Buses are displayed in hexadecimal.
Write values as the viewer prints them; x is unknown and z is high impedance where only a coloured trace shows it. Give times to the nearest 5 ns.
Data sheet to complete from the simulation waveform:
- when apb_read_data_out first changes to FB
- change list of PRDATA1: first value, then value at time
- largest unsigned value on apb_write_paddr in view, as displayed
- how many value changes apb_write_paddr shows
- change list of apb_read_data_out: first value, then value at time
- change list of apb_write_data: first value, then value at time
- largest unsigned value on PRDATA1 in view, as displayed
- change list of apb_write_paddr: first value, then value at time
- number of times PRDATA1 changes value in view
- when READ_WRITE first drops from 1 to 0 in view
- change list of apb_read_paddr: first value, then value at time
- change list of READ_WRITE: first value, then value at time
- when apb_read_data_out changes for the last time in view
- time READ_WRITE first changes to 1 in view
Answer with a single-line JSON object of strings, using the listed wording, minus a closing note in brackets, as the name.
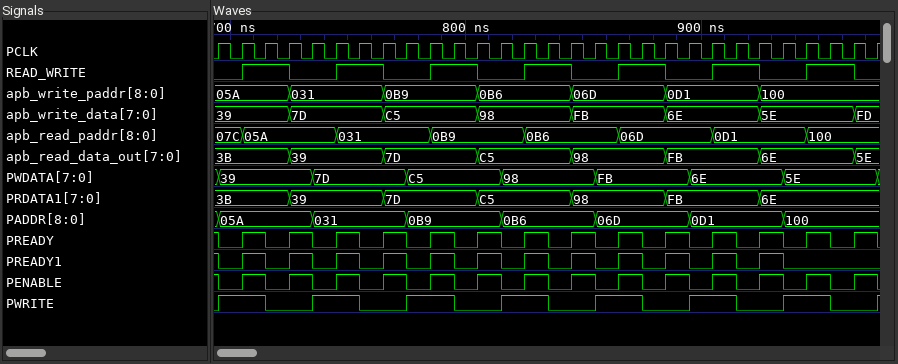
{"when apb_read_data_out first changes to FB": "885 ns", "change list of PRDATA1: first value, then value at time": "3B, 39 at 725 ns, 7D at 765 ns, C5 at 805 ns, 98 at 845 ns, FB at 885 ns, 6E at 925 ns", "largest unsigned value on apb_write_paddr in view, as displayed": "100", "how many value changes apb_write_paddr shows": "6", "change list of apb_read_data_out: first value, then value at time": "3B, 39 at 725 ns, 7D at 765 ns, C5 at 805 ns, 98 at 845 ns, FB at 885 ns, 6E at 925 ns, 5E at 965 ns", "change list of apb_write_data: first value, then value at time": "39, 7D at 725 ns, C5 at 765 ns, 98 at 805 ns, FB at 845 ns, 6E at 885 ns, 5E at 925 ns, FD at 965 ns", "largest unsigned value on PRDATA1 in view, as displayed": "FB", "change list of apb_write_paddr: first value, then value at time": "05A, 031 at 725 ns, 0B9 at 765 ns, 0B6 at 805 ns, 06D at 845 ns, 0D1 at 885 ns, 100 at 925 ns", "number of times PRDATA1 changes value in view": "6", "when READ_WRITE first drops from 1 to 0 in view": "725 ns", "change list of apb_read_paddr: first value, then value at time": "07C, 05A at 705 ns, 031 at 745 ns, 0B9 at 785 ns, 0B6 at 825 ns, 06D at 865 ns, 0D1 at 905 ns, 100 at 945 ns", "change list of READ_WRITE: first value, then value at time": "0, 1 at 705 ns, 0 at 725 ns, 1 at 745 ns, 0 at 765 ns, 1 at 785 ns, 0 at 805 ns, 1 at 825 ns, 0 at 845 ns, 1 at 865 ns, 0 at 885 ns, 1 at 905 ns, 0 at 925 ns, 1 at 945 ns, 0 at 965 ns", "when apb_read_data_out changes for the last time in view": "965 ns", "time READ_WRITE first changes to 1 in view": "705 ns"}
